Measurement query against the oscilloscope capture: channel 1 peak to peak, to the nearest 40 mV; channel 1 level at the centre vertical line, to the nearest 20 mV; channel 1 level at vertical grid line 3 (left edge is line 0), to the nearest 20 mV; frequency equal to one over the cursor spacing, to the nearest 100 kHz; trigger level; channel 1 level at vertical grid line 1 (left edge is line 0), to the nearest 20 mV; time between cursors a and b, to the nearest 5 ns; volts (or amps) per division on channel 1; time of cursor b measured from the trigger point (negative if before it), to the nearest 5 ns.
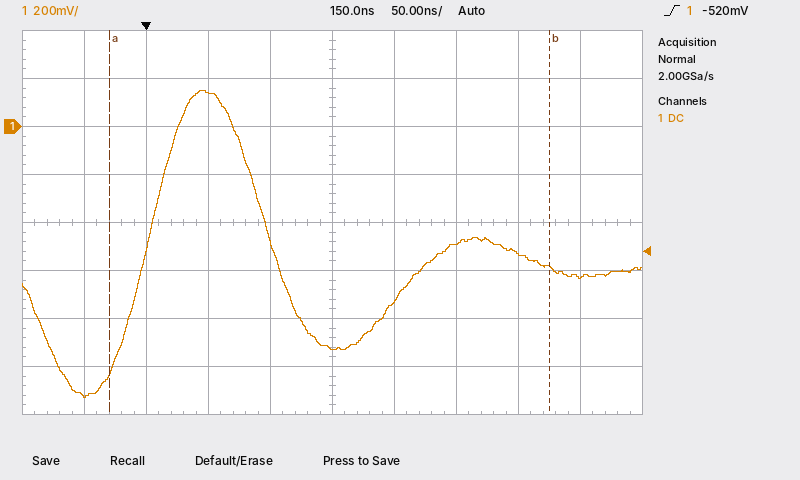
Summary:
1.28 V
-920 mV
140 mV
2.8 MHz
-520 mV
-1.12 V
355 ns
200 mV
+325 ns
